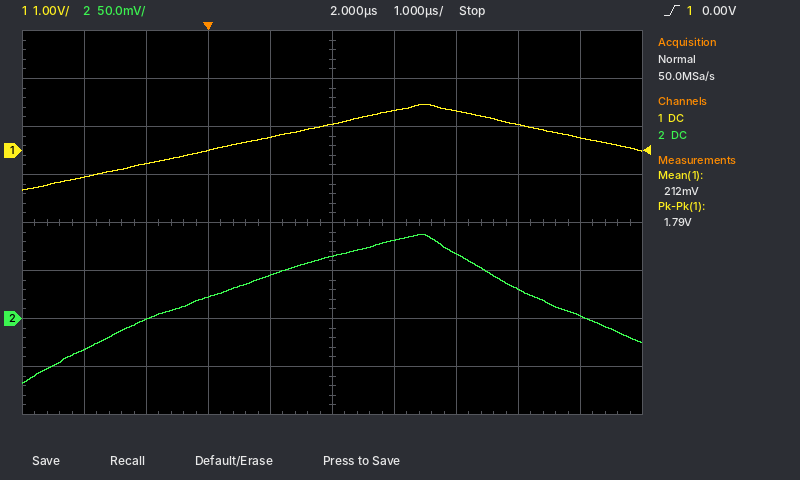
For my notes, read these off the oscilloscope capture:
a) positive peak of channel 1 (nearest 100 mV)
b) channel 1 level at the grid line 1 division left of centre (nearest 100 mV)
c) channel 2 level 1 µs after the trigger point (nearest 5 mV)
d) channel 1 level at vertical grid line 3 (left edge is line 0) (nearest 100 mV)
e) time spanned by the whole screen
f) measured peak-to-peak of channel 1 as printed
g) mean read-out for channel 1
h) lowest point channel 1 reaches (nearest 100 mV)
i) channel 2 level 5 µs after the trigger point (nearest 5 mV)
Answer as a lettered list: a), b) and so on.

a) 1.0 V
b) 300 mV
c) 45 mV
d) 0.0 V
e) 10 µs
f) 1.79 V
g) 212 mV
h) -800 mV
i) 30 mV
